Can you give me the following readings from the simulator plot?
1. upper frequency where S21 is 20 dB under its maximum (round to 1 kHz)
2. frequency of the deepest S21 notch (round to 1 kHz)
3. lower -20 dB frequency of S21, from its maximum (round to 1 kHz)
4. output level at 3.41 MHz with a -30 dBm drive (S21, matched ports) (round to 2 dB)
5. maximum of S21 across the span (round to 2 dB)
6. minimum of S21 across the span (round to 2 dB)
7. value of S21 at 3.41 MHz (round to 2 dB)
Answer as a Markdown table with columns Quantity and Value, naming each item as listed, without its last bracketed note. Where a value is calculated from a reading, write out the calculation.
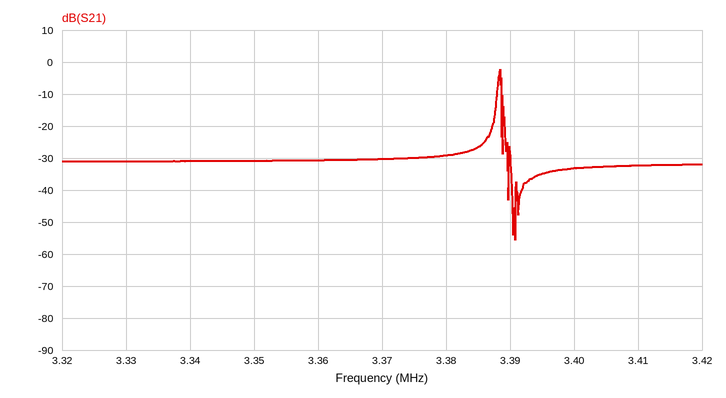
| Quantity | Value |
|---|---|
| upper frequency where S21 is 20 dB under its maximum | 3.389 MHz |
| frequency of the deepest S21 notch | 3.391 MHz |
| lower -20 dB frequency of S21, from its maximum | 3.387 MHz |
| output level at 3.41 MHz with a -30 dBm drive (S21, matched ports) | -30 dBm + (-32 dB) = -62 dBm |
| maximum of S21 across the span | -2 dB |
| minimum of S21 across the span | -56 dB |
| value of S21 at 3.41 MHz | -32 dB |
